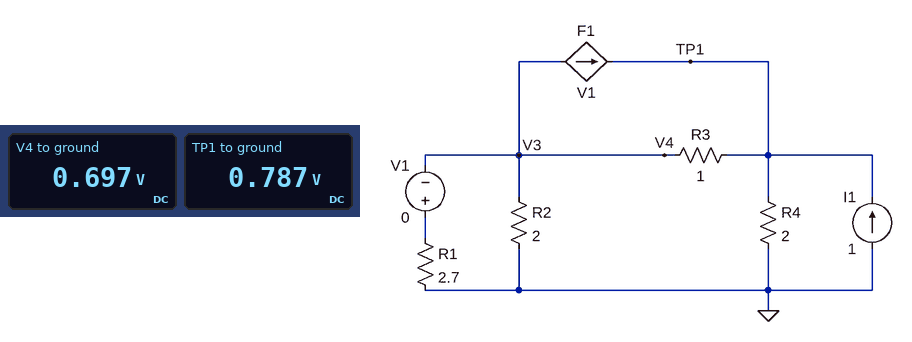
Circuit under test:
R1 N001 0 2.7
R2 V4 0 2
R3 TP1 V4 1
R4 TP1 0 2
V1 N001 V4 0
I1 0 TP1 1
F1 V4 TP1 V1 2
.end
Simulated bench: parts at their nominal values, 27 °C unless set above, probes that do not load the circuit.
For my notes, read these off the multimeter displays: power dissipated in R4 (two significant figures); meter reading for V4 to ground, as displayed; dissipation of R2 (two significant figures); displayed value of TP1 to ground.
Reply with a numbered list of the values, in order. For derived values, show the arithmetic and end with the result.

1. (787 mV)^2 / 2 Ω = 310 mW
2. 0.697 V
3. (697 mV)^2 / 2 Ω = 240 mW
4. 0.787 V
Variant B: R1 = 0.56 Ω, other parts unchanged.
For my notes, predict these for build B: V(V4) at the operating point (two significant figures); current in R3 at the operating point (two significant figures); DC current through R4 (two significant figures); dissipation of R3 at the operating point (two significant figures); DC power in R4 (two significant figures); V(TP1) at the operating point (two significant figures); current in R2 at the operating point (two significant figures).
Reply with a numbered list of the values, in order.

1. 470 mV
2. 600 mA
3. 67 mA
4. 360 mW
5. 8.9 mW
6. -130 mV
7. 230 mA
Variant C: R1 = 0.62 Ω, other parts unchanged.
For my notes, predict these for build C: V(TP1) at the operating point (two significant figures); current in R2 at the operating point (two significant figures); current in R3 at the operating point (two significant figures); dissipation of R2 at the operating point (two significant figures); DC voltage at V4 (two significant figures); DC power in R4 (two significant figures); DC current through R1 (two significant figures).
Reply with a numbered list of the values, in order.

1. -55 mV
2. 240 mA
3. 540 mA
4. 120 mW
5. 490 mV
6. 1.5 mW
7. 780 mA
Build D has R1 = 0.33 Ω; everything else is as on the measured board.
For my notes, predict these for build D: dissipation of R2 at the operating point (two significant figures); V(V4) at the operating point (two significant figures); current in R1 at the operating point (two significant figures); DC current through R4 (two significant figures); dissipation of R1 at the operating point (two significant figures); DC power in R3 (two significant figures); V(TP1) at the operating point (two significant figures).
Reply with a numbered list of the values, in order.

1. 65 mW
2. 360 mV
3. 1.1 A
4. 280 mA
5. 400 mW
6. 840 mW
7. -550 mV
